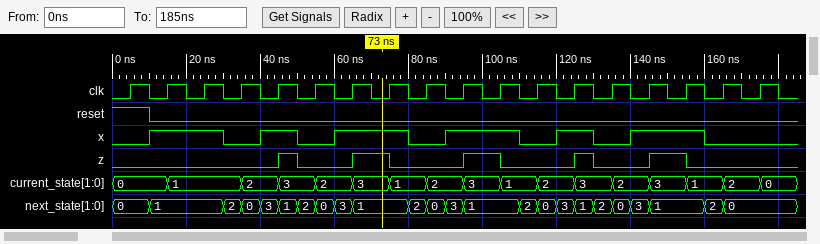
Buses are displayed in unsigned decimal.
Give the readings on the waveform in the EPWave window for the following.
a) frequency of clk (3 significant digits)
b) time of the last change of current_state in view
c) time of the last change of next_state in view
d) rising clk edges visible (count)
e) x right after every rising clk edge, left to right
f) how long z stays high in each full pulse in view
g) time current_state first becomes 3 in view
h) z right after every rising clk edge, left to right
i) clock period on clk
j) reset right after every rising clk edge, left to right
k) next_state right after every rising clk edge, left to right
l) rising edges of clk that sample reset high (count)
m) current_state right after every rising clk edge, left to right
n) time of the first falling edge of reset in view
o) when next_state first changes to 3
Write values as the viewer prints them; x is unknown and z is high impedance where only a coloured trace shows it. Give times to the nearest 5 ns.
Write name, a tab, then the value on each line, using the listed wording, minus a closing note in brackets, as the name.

frequency of clk	100 MHz
time of the last change of current_state in view	175 ns
time of the last change of next_state in view	165 ns
rising clk edges visible	18
x right after every rising clk edge, left to right	0 1 1 0 1 0 1 1 0 1 1 0 1 0 1 1 0 0
how long z stays high in each full pulse in view	5 ns, 10 ns, 10 ns, 5 ns, 10 ns
time current_state first becomes 3 in view	45 ns
z right after every rising clk edge, left to right	0 0 0 0 1 0 1 0 0 1 0 0 1 0 1 0 0 0
clock period on clk	10 ns
reset right after every rising clk edge, left to right	1 0 0 0 0 0 0 0 0 0 0 0 0 0 0 0 0 0
next_state right after every rising clk edge, left to right	0, 1, 1, 0, 1, 0, 1, 1, 0, 1, 1, 0, 1, 0, 1, 1, 0, 0
rising edges of clk that sample reset high	1
current_state right after every rising clk edge, left to right	0, 1, 1, 2, 3, 2, 3, 1, 2, 3, 1, 2, 3, 2, 3, 1, 2, 0
time of the first falling edge of reset in view	10 ns
when next_state first changes to 3	40 ns
